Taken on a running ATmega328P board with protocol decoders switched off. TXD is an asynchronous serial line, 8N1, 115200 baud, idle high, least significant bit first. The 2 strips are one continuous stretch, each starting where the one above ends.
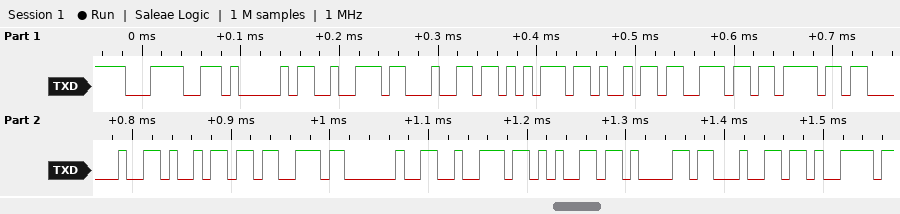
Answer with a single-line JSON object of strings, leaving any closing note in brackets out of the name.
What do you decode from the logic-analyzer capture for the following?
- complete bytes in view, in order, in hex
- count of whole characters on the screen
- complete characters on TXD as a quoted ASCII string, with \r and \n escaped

{"complete bytes in view, in order, in hex": "0x3C 0x41 0x72 0x64 0x75 0x69 0x6E 0x6F 0x20 0x69 0x73 0x20 0x72 0x65 0x61 0x64 0x79", "count of whole characters on the screen": "17", "complete characters on TXD as a quoted ASCII string, with \\r and \\n escaped": "\"<Arduino is ready\""}
